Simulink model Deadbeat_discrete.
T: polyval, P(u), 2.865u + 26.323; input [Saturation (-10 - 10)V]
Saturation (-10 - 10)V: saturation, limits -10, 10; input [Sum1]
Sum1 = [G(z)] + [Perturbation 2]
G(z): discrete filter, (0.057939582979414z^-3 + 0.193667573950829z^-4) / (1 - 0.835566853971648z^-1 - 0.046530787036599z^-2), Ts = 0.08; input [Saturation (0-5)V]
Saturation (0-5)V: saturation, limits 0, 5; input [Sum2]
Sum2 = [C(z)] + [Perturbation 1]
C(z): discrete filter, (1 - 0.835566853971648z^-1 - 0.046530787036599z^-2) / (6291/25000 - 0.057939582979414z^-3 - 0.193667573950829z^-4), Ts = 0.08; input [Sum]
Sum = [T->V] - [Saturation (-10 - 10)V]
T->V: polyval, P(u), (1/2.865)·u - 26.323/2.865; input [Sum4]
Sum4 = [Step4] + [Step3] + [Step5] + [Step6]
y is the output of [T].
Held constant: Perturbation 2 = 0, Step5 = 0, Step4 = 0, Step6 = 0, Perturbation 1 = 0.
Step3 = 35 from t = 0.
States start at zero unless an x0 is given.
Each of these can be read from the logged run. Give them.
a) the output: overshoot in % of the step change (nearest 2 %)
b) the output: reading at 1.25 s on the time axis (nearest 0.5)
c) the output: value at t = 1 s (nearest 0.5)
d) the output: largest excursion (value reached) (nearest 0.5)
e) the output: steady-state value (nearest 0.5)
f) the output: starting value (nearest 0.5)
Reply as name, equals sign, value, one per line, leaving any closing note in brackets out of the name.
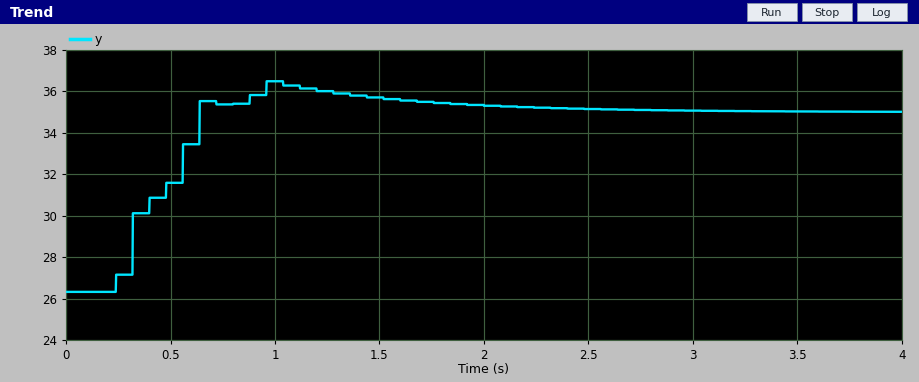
the output: overshoot in % of the step change = 18 %
the output: reading at 1.25 s on the time axis = 36.0
the output: value at t = 1 s = 36.5
the output: largest excursion (value reached) = 36.5
the output: steady-state value = 35.0
the output: starting value = 26.5
